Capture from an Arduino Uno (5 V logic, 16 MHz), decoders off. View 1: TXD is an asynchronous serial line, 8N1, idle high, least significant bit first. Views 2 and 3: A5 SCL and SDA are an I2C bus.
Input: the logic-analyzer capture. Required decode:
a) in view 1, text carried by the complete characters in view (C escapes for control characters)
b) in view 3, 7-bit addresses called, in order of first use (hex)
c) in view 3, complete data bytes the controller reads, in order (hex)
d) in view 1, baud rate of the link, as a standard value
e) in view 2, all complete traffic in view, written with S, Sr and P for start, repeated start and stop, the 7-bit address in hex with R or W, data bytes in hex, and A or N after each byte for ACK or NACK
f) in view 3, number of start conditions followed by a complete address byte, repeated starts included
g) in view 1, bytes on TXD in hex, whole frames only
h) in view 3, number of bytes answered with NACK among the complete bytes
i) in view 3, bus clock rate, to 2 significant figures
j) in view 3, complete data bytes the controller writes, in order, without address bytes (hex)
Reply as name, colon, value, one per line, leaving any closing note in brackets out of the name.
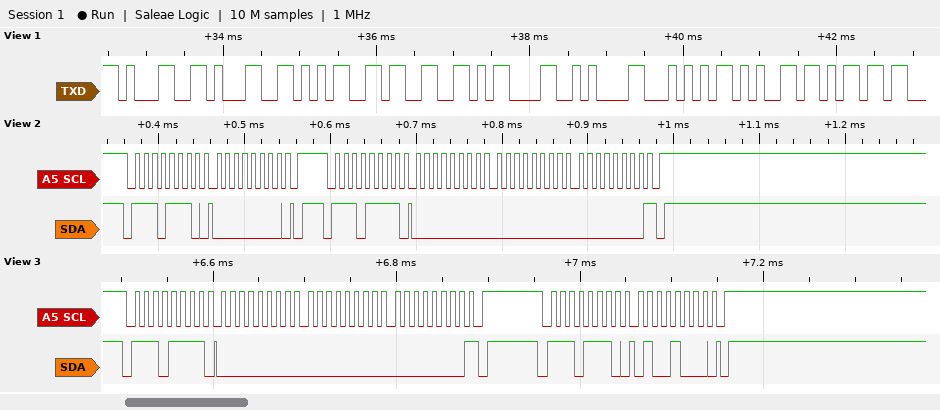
in view 1, text carried by the complete characters in view: "1153\r\nTem"
in view 3, 7-bit addresses called, in order of first use: 0x77
in view 3, complete data bytes the controller reads, in order: 00 00 00
in view 1, baud rate of the link, as a standard value: 9600 baud
in view 2, all complete traffic in view, written with S, Sr and P for start, repeated start and stop, the 7-bit address in hex with R or W, data bytes in hex, and A or N after each byte for ACK or NACK: S 77W A 00 A P S 77R A 00 A 00 A 00 N P
in view 3, number of start conditions followed by a complete address byte, repeated starts included: 2
in view 1, bytes on TXD in hex, whole frames only: 31 31 35 33 0D 0A 54 65 6D
in view 3, number of bytes answered with NACK among the complete bytes: 1
in view 3, bus clock rate, to 2 significant figures: 100 kHz
in view 3, complete data bytes the controller writes, in order, without address bytes: 48
